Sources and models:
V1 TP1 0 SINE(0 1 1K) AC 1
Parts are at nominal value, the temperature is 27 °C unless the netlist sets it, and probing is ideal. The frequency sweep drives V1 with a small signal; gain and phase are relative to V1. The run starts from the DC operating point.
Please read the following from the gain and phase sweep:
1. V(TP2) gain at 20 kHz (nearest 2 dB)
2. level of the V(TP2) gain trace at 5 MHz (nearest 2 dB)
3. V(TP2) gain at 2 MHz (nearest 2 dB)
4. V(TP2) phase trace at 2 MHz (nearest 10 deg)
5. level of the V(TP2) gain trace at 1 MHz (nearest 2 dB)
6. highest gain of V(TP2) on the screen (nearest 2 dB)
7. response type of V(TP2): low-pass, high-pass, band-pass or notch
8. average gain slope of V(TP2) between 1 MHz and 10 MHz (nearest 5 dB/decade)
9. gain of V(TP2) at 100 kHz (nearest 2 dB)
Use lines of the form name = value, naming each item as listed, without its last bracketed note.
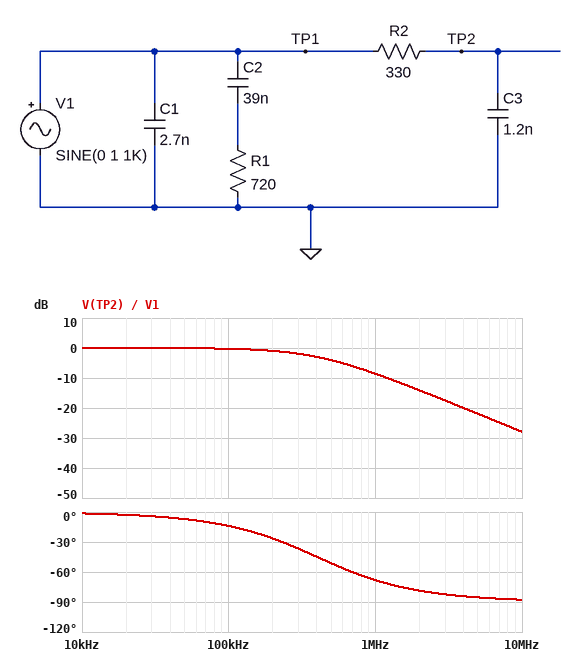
V(TP2) gain at 20 kHz = 0 dB
level of the V(TP2) gain trace at 5 MHz = -22 dB
V(TP2) gain at 2 MHz = -14 dB
V(TP2) phase trace at 2 MHz = -80 deg
level of the V(TP2) gain trace at 1 MHz = -8 dB
highest gain of V(TP2) on the screen = 0 dB
response type of V(TP2): low-pass, high-pass, band-pass or notch = low-pass
average gain slope of V(TP2) between 1 MHz and 10 MHz = -20 dB/decade
gain of V(TP2) at 100 kHz = 0 dB
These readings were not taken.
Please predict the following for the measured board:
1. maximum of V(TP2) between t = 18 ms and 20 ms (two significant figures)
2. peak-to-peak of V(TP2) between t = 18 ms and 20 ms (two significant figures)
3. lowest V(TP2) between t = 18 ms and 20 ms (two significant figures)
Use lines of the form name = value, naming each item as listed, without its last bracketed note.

maximum of V(TP2) between t = 18 ms and 20 ms = 1.0 V
peak-to-peak of V(TP2) between t = 18 ms and 20 ms = 2.0 V
lowest V(TP2) between t = 18 ms and 20 ms = -1.0 V
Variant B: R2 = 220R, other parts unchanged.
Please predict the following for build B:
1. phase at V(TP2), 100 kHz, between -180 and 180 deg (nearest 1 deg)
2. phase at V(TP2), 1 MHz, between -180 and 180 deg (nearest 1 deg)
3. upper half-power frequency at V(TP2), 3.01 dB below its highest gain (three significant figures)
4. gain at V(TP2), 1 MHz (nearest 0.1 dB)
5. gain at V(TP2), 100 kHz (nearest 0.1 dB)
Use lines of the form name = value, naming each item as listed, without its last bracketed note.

phase at V(TP2), 100 kHz, between -180 and 180 deg = -9 deg
phase at V(TP2), 1 MHz, between -180 and 180 deg = -59 deg
upper half-power frequency at V(TP2), 3.01 dB below its highest gain = 603 kHz
gain at V(TP2), 1 MHz = -5.7 dB
gain at V(TP2), 100 kHz = -0.1 dB
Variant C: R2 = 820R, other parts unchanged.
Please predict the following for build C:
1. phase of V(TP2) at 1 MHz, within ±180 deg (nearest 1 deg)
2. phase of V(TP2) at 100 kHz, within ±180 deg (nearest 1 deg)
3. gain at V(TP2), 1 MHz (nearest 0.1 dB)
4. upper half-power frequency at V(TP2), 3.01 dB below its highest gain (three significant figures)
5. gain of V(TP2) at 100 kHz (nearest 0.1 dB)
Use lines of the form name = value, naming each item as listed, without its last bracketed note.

phase of V(TP2) at 1 MHz, within ±180 deg = -81 deg
phase of V(TP2) at 100 kHz, within ±180 deg = -32 deg
gain at V(TP2), 1 MHz = -15.9 dB
upper half-power frequency at V(TP2), 3.01 dB below its highest gain = 162 kHz
gain of V(TP2) at 100 kHz = -1.4 dB
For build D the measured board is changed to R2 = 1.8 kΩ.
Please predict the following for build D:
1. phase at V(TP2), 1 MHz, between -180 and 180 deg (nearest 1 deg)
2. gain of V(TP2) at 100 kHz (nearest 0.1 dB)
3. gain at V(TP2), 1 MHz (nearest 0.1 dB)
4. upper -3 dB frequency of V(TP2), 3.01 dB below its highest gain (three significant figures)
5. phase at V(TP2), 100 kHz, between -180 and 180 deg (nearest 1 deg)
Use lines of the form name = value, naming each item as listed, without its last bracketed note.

phase at V(TP2), 1 MHz, between -180 and 180 deg = -86 deg
gain of V(TP2) at 100 kHz = -4.5 dB
gain at V(TP2), 1 MHz = -22.7 dB
upper -3 dB frequency of V(TP2), 3.01 dB below its highest gain = 73.7 kHz
phase at V(TP2), 100 kHz, between -180 and 180 deg = -54 deg
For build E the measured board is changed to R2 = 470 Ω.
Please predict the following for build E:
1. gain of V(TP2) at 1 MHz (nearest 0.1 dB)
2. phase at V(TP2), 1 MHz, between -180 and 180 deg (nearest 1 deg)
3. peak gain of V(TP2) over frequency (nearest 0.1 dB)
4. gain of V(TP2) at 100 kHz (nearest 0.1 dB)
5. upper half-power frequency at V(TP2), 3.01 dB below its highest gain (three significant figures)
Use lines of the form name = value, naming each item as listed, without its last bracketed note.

gain of V(TP2) at 1 MHz = -11.3 dB
phase at V(TP2), 1 MHz, between -180 and 180 deg = -74 deg
peak gain of V(TP2) over frequency = 0 dB
gain of V(TP2) at 100 kHz = -0.5 dB
upper half-power frequency at V(TP2), 3.01 dB below its highest gain = 282 kHz
